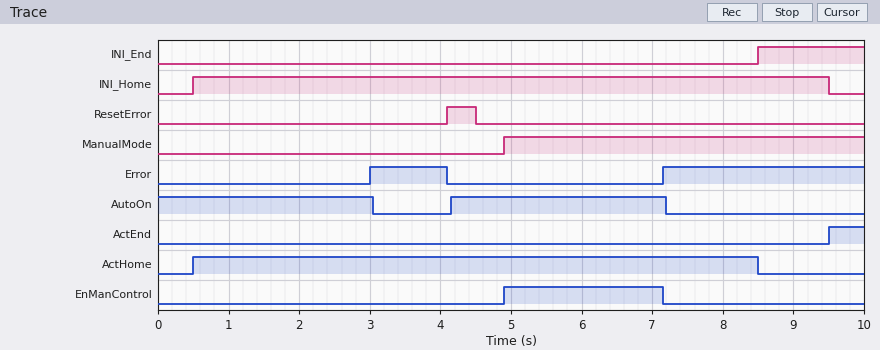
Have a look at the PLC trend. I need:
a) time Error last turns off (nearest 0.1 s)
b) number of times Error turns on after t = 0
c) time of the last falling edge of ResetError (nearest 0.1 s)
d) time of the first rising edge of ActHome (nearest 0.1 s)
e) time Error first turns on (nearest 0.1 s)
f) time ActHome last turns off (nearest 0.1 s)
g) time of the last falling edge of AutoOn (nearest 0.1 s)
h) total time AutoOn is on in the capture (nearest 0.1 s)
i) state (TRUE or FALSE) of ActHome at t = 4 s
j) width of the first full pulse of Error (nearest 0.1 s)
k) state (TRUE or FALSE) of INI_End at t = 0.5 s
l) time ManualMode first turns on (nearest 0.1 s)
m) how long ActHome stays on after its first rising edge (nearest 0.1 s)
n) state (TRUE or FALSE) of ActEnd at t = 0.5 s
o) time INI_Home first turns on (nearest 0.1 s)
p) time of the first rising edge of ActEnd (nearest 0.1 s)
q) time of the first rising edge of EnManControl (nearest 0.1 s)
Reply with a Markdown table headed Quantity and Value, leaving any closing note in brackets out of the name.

| Quantity | Value |
|---|---|
| time Error last turns off | 4.1 s |
| number of times Error turns on after t = 0 | 2 |
| time of the last falling edge of ResetError | 4.5 s |
| time of the first rising edge of ActHome | 0.5 s |
| time Error first turns on | 3.0 s |
| time ActHome last turns off | 8.5 s |
| time of the last falling edge of AutoOn | 7.2 s |
| total time AutoOn is on in the capture | 6.1 s |
| state (TRUE or FALSE) of ActHome at t = 4 s | TRUE |
| width of the first full pulse of Error | 1.1 s |
| state (TRUE or FALSE) of INI_End at t = 0.5 s | FALSE |
| time ManualMode first turns on | 4.9 s |
| how long ActHome stays on after its first rising edge | 8.0 s |
| state (TRUE or FALSE) of ActEnd at t = 0.5 s | FALSE |
| time INI_Home first turns on | 0.5 s |
| time of the first rising edge of ActEnd | 9.5 s |
| time of the first rising edge of EnManControl | 4.9 s |
